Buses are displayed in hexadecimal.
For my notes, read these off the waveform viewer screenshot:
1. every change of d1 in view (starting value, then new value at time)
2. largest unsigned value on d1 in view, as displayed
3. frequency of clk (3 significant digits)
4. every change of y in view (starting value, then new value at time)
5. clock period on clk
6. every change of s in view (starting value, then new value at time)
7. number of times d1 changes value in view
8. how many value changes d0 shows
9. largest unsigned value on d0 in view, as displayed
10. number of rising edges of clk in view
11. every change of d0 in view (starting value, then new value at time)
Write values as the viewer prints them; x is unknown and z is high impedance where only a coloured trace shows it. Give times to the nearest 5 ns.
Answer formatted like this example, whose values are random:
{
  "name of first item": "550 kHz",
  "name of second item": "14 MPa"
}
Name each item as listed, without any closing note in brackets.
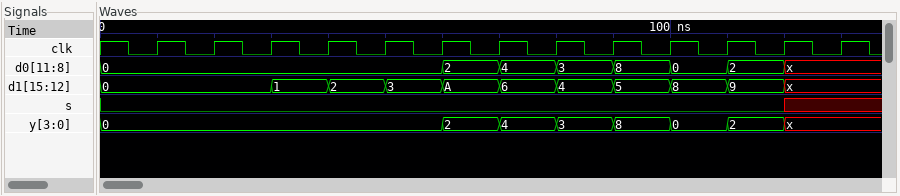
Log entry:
{
  "every change of d1 in view": "0, 1 at 30 ns, 2 at 40 ns, 3 at 50 ns, A at 60 ns, 6 at 70 ns, 4 at 80 ns, 5 at 90 ns, 8 at 100 ns, 9 at 110 ns, x at 120 ns",
  "largest unsigned value on d1 in view, as displayed": "A",
  "frequency of clk": "100 MHz",
  "every change of y in view": "0, 2 at 60 ns, 4 at 70 ns, 3 at 80 ns, 8 at 90 ns, 0 at 100 ns, 2 at 110 ns, x at 120 ns",
  "clock period on clk": "10 ns",
  "every change of s in view": "0, x at 120 ns",
  "number of times d1 changes value in view": "10",
  "how many value changes d0 shows": "7",
  "largest unsigned value on d0 in view, as displayed": "8",
  "number of rising edges of clk in view": "13",
  "every change of d0 in view": "0, 2 at 60 ns, 4 at 70 ns, 3 at 80 ns, 8 at 90 ns, 0 at 100 ns, 2 at 110 ns, x at 120 ns"
}
